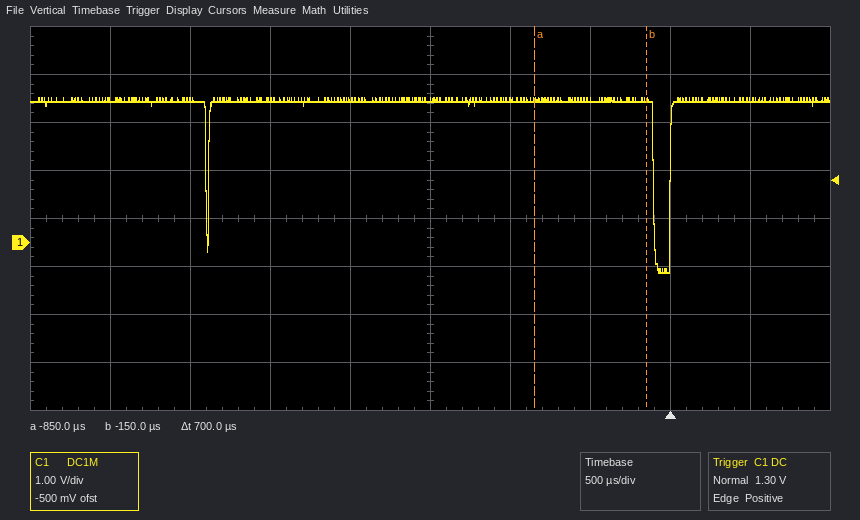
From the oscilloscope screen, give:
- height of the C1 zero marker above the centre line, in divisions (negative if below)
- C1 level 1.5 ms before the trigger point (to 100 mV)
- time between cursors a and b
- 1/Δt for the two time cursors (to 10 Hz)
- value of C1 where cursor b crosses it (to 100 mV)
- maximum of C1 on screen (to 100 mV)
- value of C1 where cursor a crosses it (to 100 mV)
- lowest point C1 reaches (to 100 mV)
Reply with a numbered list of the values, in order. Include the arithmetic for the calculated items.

1. -0.5 div
2. 3.0 V
3. 700 µs
4. 1 / 700 µs ≈ 1.43 kHz
5. 3.0 V
6. 3.0 V
7. 3.0 V
8. -600 mV
